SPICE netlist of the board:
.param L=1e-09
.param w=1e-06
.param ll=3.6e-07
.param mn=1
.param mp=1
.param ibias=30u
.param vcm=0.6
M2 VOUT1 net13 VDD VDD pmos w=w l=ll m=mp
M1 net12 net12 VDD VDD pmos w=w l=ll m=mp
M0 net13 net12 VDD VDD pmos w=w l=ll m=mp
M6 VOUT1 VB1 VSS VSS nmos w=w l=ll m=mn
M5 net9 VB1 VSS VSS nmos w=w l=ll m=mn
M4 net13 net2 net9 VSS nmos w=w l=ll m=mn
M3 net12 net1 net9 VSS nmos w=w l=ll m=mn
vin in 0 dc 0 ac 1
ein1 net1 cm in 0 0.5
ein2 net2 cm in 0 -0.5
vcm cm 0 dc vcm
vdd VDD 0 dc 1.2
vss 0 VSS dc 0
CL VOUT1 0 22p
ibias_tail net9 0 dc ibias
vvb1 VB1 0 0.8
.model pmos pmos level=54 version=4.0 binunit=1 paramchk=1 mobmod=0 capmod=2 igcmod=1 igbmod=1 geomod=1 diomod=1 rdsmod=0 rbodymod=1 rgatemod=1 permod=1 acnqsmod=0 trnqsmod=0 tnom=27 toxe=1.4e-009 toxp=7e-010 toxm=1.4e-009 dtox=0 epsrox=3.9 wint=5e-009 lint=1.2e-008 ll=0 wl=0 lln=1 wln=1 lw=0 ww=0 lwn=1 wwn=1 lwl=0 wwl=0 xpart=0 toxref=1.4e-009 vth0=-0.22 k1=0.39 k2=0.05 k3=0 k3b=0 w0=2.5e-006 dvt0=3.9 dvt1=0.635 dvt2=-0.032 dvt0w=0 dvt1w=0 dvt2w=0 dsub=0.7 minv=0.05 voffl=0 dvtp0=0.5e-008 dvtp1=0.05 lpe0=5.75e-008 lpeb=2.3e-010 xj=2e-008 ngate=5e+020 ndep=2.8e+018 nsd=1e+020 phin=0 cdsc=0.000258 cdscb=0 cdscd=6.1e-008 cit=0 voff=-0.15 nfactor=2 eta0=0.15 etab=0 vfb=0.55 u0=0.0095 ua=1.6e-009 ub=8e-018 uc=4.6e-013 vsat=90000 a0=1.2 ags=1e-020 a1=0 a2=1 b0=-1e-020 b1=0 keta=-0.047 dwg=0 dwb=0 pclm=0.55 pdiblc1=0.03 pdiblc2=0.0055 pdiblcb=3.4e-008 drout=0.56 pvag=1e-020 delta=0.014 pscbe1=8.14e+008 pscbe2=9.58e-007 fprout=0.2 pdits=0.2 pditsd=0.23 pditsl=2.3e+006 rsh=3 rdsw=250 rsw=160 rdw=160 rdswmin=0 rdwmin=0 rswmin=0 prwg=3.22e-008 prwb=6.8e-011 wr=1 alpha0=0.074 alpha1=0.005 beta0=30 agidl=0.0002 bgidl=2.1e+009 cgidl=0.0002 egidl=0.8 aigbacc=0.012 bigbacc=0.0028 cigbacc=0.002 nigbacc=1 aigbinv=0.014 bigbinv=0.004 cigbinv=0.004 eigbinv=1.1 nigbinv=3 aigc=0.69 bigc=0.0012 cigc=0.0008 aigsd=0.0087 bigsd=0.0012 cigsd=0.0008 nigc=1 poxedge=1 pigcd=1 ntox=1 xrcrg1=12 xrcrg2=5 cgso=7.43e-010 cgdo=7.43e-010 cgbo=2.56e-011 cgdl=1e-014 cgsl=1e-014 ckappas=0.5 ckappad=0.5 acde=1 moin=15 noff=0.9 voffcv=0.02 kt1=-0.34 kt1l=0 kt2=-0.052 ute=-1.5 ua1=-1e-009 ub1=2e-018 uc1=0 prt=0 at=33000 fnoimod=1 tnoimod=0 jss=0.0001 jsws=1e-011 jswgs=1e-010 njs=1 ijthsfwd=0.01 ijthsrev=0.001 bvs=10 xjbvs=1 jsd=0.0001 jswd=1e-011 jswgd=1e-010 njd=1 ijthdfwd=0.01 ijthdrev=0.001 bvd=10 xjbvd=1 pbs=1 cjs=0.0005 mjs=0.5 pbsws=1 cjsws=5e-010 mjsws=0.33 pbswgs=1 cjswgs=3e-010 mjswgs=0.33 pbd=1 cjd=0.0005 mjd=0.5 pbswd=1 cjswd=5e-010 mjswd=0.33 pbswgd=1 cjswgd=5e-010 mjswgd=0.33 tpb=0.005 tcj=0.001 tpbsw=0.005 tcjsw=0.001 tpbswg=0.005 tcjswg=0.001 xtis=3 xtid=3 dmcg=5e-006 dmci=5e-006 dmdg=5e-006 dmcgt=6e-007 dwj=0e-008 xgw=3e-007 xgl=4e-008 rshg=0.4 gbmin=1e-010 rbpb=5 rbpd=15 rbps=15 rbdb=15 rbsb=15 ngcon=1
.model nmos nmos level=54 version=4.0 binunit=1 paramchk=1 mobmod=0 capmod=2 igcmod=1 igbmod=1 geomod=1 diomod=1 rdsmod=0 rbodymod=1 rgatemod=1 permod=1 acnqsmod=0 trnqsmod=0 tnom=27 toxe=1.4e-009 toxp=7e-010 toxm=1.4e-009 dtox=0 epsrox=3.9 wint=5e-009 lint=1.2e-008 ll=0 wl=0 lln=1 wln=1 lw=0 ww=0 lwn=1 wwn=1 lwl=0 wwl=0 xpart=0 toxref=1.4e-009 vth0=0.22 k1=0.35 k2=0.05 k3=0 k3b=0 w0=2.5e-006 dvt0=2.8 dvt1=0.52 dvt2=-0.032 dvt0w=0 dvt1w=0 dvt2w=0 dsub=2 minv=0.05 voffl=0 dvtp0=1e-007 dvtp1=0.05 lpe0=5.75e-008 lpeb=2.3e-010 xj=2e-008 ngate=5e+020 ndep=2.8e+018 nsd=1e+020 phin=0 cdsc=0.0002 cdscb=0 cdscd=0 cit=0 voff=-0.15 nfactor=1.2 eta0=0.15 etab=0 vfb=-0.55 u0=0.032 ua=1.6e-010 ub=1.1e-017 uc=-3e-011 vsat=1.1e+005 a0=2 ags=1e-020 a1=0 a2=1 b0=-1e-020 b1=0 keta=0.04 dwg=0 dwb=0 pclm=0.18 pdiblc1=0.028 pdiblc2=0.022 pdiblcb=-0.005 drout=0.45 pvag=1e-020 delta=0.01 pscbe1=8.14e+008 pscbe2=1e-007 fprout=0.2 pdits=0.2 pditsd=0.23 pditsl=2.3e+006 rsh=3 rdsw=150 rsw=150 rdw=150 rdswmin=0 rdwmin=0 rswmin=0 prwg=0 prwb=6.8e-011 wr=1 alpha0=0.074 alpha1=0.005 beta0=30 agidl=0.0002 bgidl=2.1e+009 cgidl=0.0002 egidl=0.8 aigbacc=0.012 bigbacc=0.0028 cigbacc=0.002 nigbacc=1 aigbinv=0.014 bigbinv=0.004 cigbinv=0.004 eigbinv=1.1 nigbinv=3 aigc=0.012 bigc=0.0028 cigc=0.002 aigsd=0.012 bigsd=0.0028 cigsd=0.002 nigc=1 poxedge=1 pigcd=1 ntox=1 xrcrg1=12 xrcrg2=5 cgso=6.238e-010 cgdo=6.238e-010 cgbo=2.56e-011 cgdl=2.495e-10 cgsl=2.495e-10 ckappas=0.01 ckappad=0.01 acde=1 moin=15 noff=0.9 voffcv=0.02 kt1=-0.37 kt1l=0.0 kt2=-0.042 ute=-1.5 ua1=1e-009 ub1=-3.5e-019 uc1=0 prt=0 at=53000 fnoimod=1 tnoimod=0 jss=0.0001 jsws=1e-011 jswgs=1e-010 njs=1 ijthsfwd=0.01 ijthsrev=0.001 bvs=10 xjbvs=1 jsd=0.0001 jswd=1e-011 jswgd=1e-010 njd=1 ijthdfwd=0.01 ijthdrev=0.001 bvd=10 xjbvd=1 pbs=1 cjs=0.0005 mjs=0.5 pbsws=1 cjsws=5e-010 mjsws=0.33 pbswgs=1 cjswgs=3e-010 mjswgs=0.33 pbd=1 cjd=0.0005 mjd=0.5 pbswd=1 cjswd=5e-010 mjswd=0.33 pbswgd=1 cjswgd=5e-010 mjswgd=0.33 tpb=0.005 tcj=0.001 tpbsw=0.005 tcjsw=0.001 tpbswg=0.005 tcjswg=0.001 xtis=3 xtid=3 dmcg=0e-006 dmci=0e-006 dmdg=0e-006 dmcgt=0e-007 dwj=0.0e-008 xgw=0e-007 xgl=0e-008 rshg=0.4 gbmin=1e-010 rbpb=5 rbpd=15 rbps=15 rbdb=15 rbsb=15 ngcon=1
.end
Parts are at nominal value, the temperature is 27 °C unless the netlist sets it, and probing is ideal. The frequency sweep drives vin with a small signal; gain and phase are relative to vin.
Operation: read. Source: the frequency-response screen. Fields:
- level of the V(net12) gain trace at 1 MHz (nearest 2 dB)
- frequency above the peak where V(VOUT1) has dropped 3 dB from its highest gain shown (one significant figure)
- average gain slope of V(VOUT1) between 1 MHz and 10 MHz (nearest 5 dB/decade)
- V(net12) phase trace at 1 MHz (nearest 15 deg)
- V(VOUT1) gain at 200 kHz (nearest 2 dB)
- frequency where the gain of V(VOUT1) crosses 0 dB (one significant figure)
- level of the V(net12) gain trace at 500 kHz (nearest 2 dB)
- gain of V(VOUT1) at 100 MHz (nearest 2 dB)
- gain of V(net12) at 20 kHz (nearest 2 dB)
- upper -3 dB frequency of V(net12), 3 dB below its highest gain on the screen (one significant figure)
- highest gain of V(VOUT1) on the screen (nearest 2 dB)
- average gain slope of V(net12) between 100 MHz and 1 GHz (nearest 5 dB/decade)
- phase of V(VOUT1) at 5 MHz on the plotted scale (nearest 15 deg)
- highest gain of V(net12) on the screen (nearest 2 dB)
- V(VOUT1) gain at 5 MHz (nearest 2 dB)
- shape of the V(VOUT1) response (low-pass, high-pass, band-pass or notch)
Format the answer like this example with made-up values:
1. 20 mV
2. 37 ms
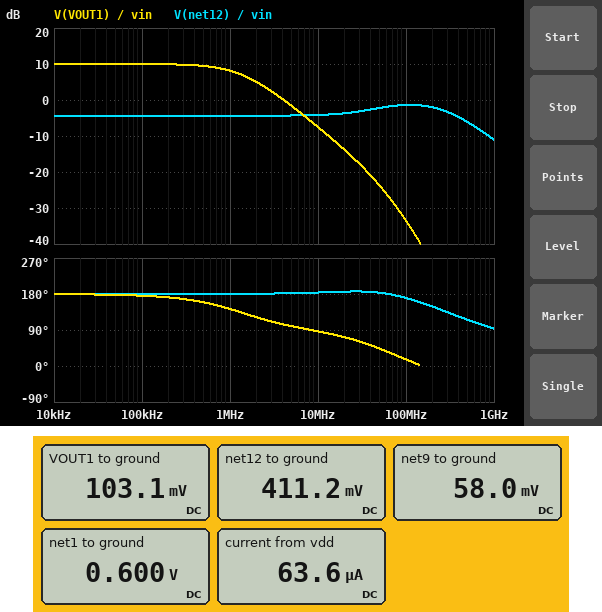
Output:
1. -4 dB
2. 1 MHz
3. -15 dB/decade
4. 180 deg
5. 10 dB
6. 4 MHz
7. -4 dB
8. -34 dB
9. -4 dB
10. 400 MHz
11. 10 dB
12. -10 dB/decade
13. 105 deg
14. -2 dB
15. -2 dB
16. low-pass
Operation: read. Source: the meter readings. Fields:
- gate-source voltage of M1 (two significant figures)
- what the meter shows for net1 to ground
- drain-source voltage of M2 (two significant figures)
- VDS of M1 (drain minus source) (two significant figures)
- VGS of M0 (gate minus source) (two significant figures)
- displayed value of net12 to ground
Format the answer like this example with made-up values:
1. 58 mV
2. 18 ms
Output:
1. -790 mV
2. 0.600 V
3. -1.1 V
4. -790 mV
5. -790 mV
6. 411.2 mV
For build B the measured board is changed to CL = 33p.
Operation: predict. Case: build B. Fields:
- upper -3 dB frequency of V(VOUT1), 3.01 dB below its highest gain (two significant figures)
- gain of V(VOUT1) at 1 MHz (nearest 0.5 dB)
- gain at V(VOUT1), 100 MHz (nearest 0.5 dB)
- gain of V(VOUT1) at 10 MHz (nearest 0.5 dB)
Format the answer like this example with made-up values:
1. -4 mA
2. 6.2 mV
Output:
1. 910 kHz
2. 6.5 dB
3. -37.0 dB
4. -11.0 dB
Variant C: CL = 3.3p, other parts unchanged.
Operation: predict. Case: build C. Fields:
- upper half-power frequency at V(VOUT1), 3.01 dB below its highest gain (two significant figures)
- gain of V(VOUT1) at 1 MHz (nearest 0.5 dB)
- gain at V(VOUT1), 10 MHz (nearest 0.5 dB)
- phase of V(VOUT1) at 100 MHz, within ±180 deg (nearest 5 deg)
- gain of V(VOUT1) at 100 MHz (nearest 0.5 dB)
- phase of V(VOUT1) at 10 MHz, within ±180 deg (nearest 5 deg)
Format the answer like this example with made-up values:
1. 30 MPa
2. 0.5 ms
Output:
1. 8.8 MHz
2. 10.0 dB
3. 6.5 dB
4. 20 deg
5. -17.0 dB
6. 120 deg
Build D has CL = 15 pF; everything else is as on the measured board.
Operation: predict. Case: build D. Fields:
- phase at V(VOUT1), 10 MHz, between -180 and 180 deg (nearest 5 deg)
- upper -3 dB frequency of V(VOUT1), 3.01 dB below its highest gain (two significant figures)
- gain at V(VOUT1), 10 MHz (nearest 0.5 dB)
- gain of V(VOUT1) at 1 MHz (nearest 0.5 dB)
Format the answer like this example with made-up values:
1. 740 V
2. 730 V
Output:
1. 90 deg
2. 2.0 MHz
3. -4.5 dB
4. 9.0 dB
